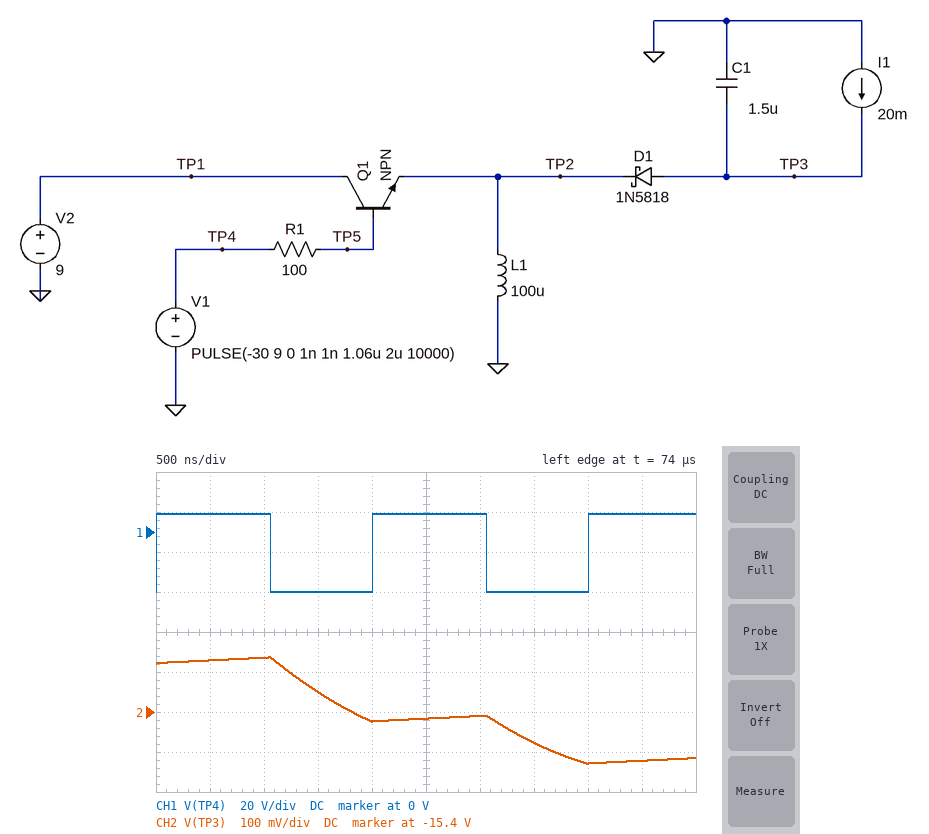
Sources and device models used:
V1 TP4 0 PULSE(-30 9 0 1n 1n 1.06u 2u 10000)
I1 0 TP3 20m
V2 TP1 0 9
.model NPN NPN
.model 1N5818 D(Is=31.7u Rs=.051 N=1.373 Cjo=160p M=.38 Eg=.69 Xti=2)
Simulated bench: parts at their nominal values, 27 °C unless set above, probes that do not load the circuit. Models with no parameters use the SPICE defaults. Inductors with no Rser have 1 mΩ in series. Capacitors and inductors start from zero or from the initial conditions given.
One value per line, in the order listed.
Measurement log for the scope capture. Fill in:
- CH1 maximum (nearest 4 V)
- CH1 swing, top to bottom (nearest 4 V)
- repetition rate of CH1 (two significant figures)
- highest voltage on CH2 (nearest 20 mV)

8 V
40 V
500 kHz
-15.26 V
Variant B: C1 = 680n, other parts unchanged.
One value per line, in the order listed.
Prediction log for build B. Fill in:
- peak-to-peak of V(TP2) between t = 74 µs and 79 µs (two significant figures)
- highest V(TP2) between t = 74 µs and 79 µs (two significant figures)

40 V
23 V
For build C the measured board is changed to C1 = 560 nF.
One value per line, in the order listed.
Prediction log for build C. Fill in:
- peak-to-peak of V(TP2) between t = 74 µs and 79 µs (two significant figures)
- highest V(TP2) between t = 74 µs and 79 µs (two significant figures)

40 V
23 V
